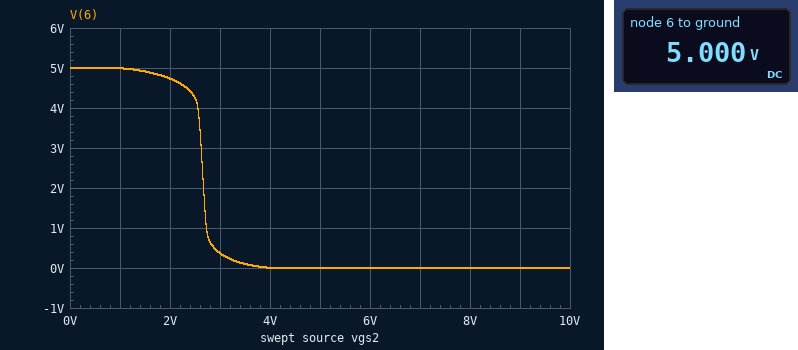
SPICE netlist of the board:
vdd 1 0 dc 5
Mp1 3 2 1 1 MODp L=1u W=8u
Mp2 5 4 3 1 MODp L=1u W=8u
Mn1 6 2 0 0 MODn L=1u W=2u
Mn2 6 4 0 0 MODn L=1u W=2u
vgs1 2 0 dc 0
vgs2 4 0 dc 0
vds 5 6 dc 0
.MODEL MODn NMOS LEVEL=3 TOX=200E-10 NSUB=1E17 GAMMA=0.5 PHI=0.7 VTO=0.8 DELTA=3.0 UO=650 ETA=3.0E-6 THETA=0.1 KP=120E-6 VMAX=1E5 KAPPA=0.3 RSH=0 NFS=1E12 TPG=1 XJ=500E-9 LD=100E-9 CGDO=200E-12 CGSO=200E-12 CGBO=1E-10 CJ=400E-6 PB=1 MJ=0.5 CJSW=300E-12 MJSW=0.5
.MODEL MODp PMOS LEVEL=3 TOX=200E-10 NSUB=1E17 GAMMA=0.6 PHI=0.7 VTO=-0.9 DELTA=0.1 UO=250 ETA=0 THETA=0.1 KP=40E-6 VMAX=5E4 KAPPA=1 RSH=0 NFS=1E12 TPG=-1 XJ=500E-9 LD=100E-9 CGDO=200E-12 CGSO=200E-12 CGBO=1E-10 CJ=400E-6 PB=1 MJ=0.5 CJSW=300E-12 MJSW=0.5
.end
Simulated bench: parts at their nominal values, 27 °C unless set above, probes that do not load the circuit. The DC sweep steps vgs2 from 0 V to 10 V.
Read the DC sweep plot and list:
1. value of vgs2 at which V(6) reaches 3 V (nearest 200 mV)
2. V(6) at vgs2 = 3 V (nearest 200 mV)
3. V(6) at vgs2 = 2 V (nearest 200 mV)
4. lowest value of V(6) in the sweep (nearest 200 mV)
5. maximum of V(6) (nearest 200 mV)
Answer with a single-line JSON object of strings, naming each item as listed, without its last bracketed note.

{"value of vgs2 at which V(6) reaches 3 V": "2.6 V", "V(6) at vgs2 = 3 V": "400 mV", "V(6) at vgs2 = 2 V": "4.8 V", "lowest value of V(6) in the sweep": "0 V", "maximum of V(6)": "5.0 V"}
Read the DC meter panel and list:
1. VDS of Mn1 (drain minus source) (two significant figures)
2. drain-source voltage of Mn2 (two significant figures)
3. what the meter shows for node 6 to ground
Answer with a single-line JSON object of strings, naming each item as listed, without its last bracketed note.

{"VDS of Mn1 (drain minus source)": "5.0 V", "drain-source voltage of Mn2": "5.0 V", "what the meter shows for node 6 to ground": "5.000 V"}
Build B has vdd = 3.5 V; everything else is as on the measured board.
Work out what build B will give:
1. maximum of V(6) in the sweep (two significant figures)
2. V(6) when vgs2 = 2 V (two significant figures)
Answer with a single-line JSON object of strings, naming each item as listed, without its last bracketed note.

{"maximum of V(6) in the sweep": "3.5 V", "V(6) when vgs2 = 2 V": "220 mV"}
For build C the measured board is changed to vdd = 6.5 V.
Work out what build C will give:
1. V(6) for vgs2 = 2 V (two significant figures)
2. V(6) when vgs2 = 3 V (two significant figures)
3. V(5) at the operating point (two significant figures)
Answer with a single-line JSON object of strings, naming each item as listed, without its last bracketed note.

{"V(6) for vgs2 = 2 V": "6.3 V", "V(6) when vgs2 = 3 V": "5.8 V", "V(5) at the operating point": "6.5 V"}
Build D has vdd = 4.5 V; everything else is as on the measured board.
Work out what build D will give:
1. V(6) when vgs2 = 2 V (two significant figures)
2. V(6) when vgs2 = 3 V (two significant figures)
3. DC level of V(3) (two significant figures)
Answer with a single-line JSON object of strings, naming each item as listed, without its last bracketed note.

{"V(6) when vgs2 = 2 V": "4.2 V", "V(6) when vgs2 = 3 V": "120 mV", "DC level of V(3)": "4.5 V"}
